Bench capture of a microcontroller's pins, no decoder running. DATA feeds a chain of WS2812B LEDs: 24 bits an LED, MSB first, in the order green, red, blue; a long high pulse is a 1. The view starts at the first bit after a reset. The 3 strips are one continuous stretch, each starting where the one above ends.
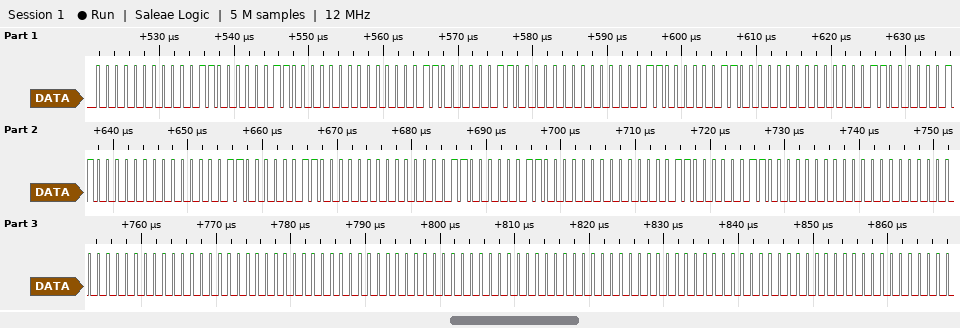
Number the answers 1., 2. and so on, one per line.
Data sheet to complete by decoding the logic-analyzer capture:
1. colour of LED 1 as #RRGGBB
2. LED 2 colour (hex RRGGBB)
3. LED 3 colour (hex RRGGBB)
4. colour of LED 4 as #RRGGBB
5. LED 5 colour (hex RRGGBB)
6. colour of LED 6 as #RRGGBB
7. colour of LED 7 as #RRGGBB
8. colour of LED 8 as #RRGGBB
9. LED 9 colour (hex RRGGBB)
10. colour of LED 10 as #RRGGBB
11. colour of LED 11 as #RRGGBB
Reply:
1. #180018
2. #180018
3. #180018
4. #180018
5. #180018
6. #180018
7. #180018
8. #000000
9. #000000
10. #000000
11. #000000
